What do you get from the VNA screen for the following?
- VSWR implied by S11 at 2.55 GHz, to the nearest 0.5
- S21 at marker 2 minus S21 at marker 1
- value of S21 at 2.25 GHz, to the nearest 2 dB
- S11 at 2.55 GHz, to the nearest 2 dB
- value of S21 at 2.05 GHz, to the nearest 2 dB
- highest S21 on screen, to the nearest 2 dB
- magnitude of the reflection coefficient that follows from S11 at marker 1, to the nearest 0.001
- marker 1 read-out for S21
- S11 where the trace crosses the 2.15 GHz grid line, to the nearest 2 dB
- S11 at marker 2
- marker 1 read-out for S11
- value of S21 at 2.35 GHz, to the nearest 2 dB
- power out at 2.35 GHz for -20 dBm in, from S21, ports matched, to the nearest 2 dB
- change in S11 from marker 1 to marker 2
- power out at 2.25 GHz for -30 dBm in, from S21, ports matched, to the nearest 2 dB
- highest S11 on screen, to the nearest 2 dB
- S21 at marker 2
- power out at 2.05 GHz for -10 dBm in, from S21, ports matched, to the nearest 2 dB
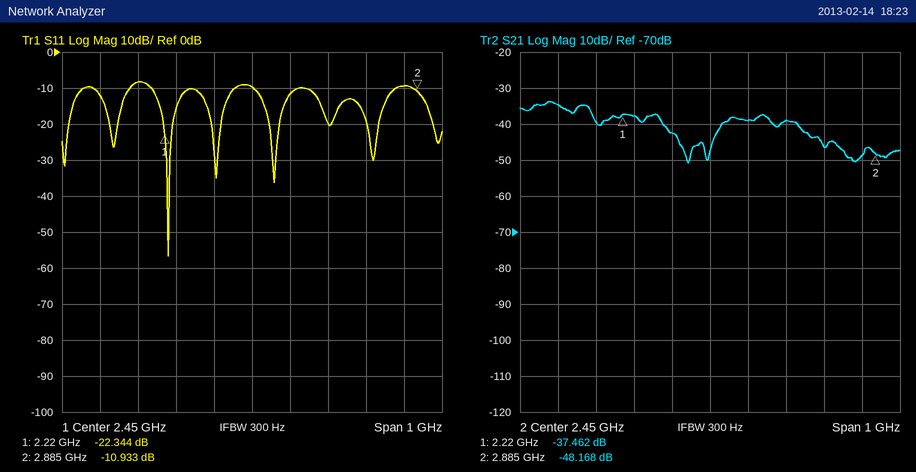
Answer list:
1.5
-10.706 dB
-38 dB
-12 dB
-34 dB
-34 dB
0.076
-37.462 dB
-8 dB
-10.933 dB
-22.344 dB
-42 dB
-62 dBm
11.411 dB
-68 dBm
-8 dB
-48.168 dB
-44 dBm
